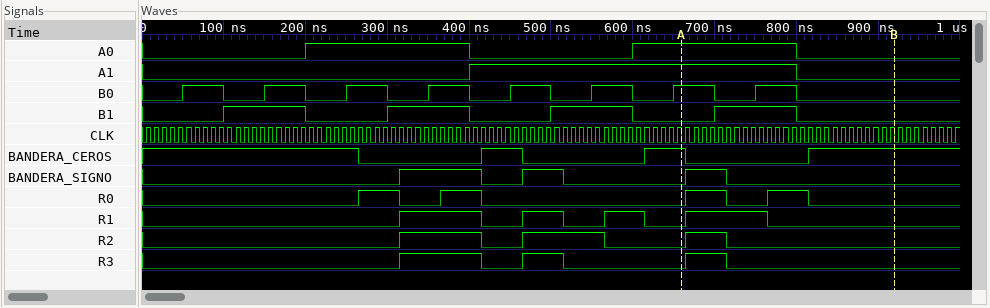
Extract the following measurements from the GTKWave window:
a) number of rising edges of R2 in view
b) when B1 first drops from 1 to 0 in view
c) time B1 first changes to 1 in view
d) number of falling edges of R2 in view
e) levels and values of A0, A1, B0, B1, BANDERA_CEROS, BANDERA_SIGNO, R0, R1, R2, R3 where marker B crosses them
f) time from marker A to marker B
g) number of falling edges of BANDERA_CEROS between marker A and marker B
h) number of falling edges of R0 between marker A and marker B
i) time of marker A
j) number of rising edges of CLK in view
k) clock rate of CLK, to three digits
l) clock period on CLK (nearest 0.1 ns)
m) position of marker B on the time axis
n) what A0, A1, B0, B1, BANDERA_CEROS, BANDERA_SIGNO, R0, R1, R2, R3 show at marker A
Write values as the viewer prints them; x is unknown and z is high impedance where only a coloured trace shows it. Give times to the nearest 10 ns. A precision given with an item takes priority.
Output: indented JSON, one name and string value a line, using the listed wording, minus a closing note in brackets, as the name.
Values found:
{
  "number of rising edges of R2 in view": "3",
  "when B1 first drops from 1 to 0 in view": "200 ns",
  "time B1 first changes to 1 in view": "100 ns",
  "number of falling edges of R2 in view": "3",
  "levels and values of A0, A1, B0, B1, BANDERA_CEROS, BANDERA_SIGNO, R0, R1, R2, R3 where marker B crosses them": "A0=0, A1=0, B0=0, B1=0, BANDERA_CEROS=1, BANDERA_SIGNO=0, R0=0, R1=0, R2=0, R3=0",
  "time from marker A to marker B": "260 ns",
  "number of falling edges of BANDERA_CEROS between marker A and marker B": "1",
  "number of falling edges of R0 between marker A and marker B": "2",
  "time of marker A": "660 ns",
  "number of rising edges of CLK in view": "100",
  "clock rate of CLK, to three digits": "100 MHz",
  "clock period on CLK": "10 ns",
  "position of marker B on the time axis": "920 ns",
  "what A0, A1, B0, B1, BANDERA_CEROS, BANDERA_SIGNO, R0, R1, R2, R3 show at marker A": "A0=1, A1=1, B0=1, B1=0, BANDERA_CEROS=1, BANDERA_SIGNO=0, R0=0, R1=0, R2=0, R3=0"
}
